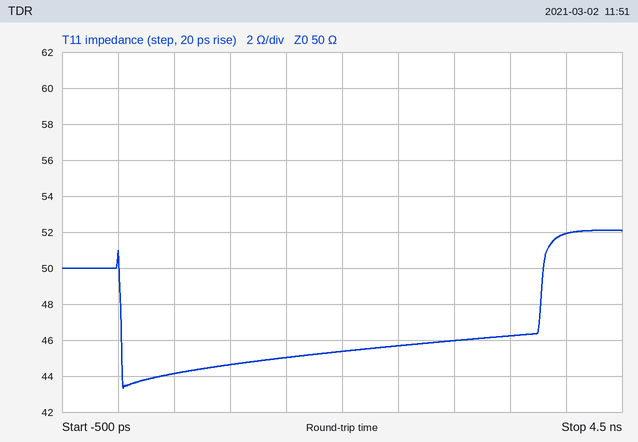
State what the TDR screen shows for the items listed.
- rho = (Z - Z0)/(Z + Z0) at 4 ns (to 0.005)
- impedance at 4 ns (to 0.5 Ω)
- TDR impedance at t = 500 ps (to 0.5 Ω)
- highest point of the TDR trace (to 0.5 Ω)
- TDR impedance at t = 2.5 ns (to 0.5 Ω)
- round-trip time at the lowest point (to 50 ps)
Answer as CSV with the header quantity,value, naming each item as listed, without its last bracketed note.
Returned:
quantity,value
rho = (Z - Z0)/(Z + Z0) at 4 ns,+0.020
impedance at 4 ns,52.0 Ω
TDR impedance at t = 500 ps,44.0 Ω
highest point of the TDR trace,52.0 Ω
TDR impedance at t = 2.5 ns,45.5 Ω
round-trip time at the lowest point,50 ps
